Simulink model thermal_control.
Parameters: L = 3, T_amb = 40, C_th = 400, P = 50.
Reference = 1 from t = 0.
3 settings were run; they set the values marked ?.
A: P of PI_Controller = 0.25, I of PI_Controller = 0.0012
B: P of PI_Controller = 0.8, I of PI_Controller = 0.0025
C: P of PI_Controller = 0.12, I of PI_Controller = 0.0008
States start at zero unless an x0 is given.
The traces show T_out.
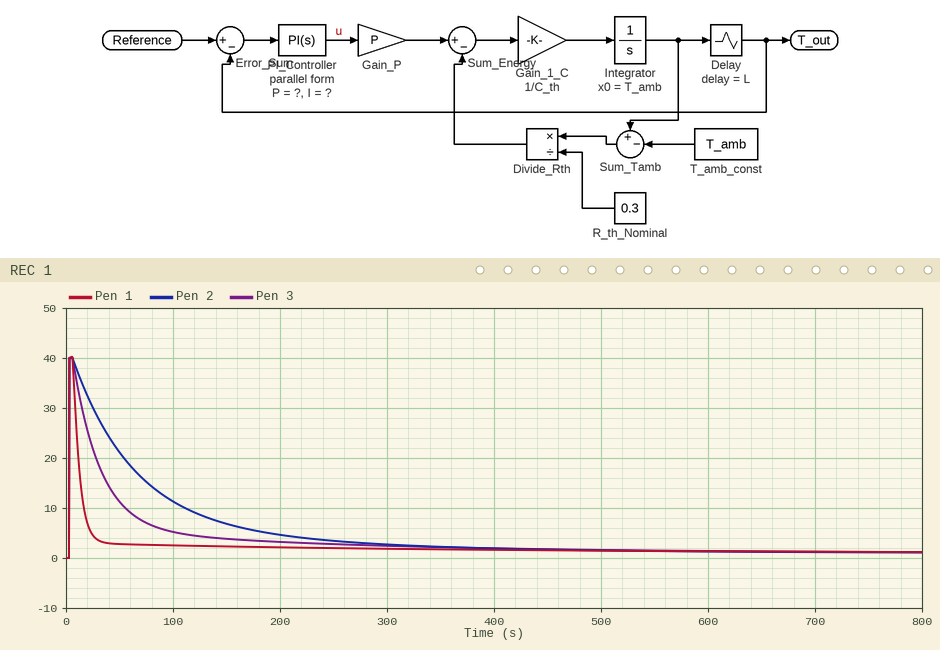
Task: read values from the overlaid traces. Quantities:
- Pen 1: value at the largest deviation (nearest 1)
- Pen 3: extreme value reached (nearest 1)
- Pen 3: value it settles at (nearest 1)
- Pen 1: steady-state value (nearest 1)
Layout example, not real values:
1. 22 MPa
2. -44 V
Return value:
1. 40
2. 40
3. 1
4. 1
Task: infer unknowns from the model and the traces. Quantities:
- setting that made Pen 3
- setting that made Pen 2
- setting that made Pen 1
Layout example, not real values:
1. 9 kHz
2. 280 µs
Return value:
1. A
2. C
3. B
